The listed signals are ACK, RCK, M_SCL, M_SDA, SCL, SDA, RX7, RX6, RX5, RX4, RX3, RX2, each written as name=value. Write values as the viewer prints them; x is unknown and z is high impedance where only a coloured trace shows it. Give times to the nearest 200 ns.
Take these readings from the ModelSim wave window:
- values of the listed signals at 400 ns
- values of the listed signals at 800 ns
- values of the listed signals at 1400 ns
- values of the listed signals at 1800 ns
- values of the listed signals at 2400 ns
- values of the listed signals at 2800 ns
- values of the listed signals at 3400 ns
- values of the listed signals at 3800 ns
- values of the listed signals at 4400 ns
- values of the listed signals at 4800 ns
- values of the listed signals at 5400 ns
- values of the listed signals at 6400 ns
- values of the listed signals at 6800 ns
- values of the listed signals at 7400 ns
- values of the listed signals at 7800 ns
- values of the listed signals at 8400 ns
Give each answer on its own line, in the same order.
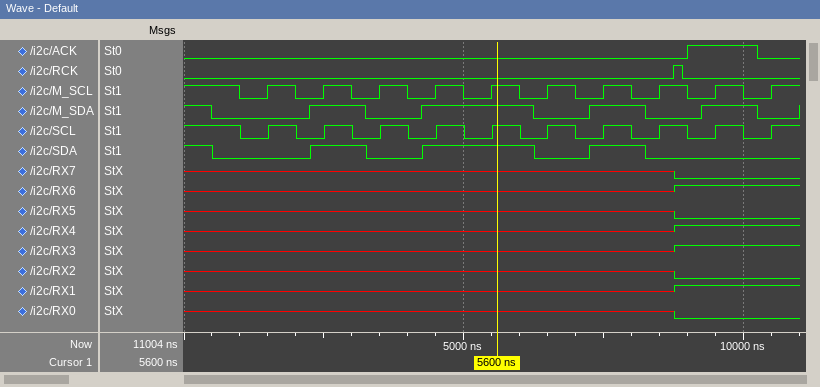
ACK=0, RCK=0, M_SCL=1, M_SDA=1, SCL=1, SDA=1, RX7=x, RX6=x, RX5=x, RX4=x, RX3=x, RX2=x
ACK=0, RCK=0, M_SCL=1, M_SDA=0, SCL=1, SDA=0, RX7=x, RX6=x, RX5=x, RX4=x, RX3=x, RX2=x
ACK=0, RCK=0, M_SCL=0, M_SDA=0, SCL=0, SDA=0, RX7=x, RX6=x, RX5=x, RX4=x, RX3=x, RX2=x
ACK=0, RCK=0, M_SCL=1, M_SDA=0, SCL=1, SDA=0, RX7=x, RX6=x, RX5=x, RX4=x, RX3=x, RX2=x
ACK=0, RCK=0, M_SCL=0, M_SDA=1, SCL=0, SDA=1, RX7=x, RX6=x, RX5=x, RX4=x, RX3=x, RX2=x
ACK=0, RCK=0, M_SCL=1, M_SDA=1, SCL=1, SDA=1, RX7=x, RX6=x, RX5=x, RX4=x, RX3=x, RX2=x
ACK=0, RCK=0, M_SCL=0, M_SDA=0, SCL=0, SDA=0, RX7=x, RX6=x, RX5=x, RX4=x, RX3=x, RX2=x
ACK=0, RCK=0, M_SCL=1, M_SDA=0, SCL=1, SDA=0, RX7=x, RX6=x, RX5=x, RX4=x, RX3=x, RX2=x
ACK=0, RCK=0, M_SCL=0, M_SDA=1, SCL=0, SDA=1, RX7=x, RX6=x, RX5=x, RX4=x, RX3=x, RX2=x
ACK=0, RCK=0, M_SCL=1, M_SDA=1, SCL=1, SDA=1, RX7=x, RX6=x, RX5=x, RX4=x, RX3=x, RX2=x
ACK=0, RCK=0, M_SCL=0, M_SDA=1, SCL=0, SDA=1, RX7=x, RX6=x, RX5=x, RX4=x, RX3=x, RX2=x
ACK=0, RCK=0, M_SCL=0, M_SDA=0, SCL=0, SDA=0, RX7=x, RX6=x, RX5=x, RX4=x, RX3=x, RX2=x
ACK=0, RCK=0, M_SCL=1, M_SDA=0, SCL=1, SDA=0, RX7=x, RX6=x, RX5=x, RX4=x, RX3=x, RX2=x
ACK=0, RCK=0, M_SCL=0, M_SDA=1, SCL=0, SDA=1, RX7=x, RX6=x, RX5=x, RX4=x, RX3=x, RX2=x
ACK=0, RCK=0, M_SCL=1, M_SDA=1, SCL=1, SDA=1, RX7=x, RX6=x, RX5=x, RX4=x, RX3=x, RX2=x
ACK=0, RCK=0, M_SCL=0, M_SDA=0, SCL=0, SDA=0, RX7=x, RX6=x, RX5=x, RX4=x, RX3=x, RX2=x
